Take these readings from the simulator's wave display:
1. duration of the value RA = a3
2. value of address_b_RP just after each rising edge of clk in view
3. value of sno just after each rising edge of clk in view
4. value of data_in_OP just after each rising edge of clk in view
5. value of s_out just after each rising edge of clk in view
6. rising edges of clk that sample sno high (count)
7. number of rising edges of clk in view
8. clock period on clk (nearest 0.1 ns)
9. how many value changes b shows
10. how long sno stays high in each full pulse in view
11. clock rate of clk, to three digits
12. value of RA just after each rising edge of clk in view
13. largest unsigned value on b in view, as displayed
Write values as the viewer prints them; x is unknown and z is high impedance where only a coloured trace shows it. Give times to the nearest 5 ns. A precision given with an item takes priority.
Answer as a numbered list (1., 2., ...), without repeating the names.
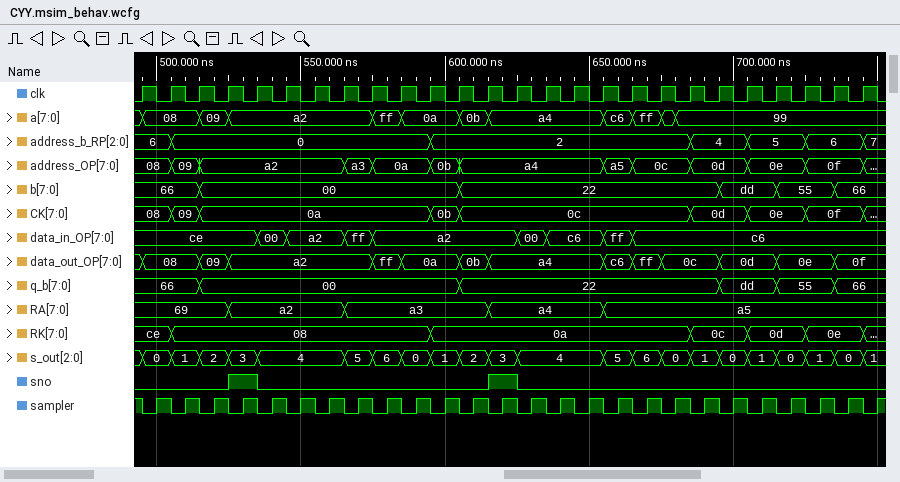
1. 50 ns
2. 6, 0, 0, 0, 0, 0, 0, 0, 0, 0, 2, 2, 2, 2, 2, 2, 2, 2, 2, 4, 4, 5, 5, 6, 6, 7
3. 0 0 0 1 0 0 0 0 0 0 0 0 1 0 0 0 0 0 0 0 0 0 0 0 0 0
4. ce, ce, ce, ce, 00, a2, a2, ff, a2, a2, a2, a2, a2, 00, c6, c6, ff, c6, c6, c6, c6, c6, c6, c6, c6, c6
5. 0, 1, 2, 3, 4, 4, 4, 5, 6, 0, 1, 2, 3, 4, 4, 4, 5, 6, 0, 1, 0, 1, 0, 1, 0, 1
6. 2
7. 26
8. 10 ns
9. 5
10. 10 ns, 10 ns
11. 100 MHz
12. 69, 69, 69, a2, a2, a2, a2, a3, a3, a3, a3, a3, a4, a4, a4, a4, a5, a5, a5, a5, a5, a5, a5, a5, a5, a5
13. dd
